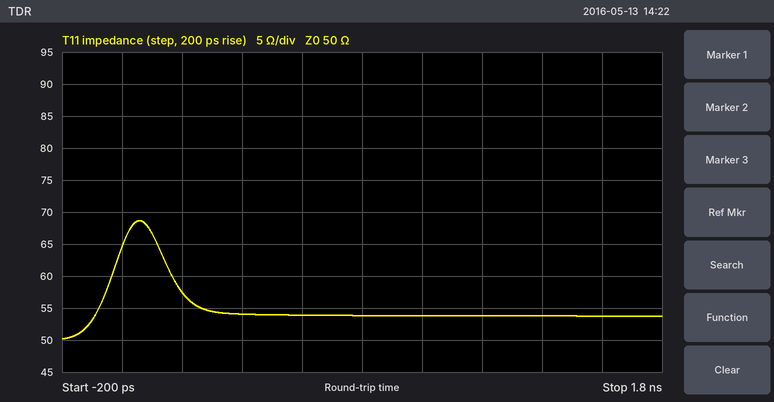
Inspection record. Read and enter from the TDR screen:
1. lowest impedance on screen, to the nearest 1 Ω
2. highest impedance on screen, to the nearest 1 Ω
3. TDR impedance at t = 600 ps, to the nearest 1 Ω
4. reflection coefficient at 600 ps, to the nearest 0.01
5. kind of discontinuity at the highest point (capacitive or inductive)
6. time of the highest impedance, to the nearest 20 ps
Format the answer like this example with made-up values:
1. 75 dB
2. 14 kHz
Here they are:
1. 50 Ω
2. 69 Ω
3. 54 Ω
4. +0.04
5. inductive
6. 60 ps
